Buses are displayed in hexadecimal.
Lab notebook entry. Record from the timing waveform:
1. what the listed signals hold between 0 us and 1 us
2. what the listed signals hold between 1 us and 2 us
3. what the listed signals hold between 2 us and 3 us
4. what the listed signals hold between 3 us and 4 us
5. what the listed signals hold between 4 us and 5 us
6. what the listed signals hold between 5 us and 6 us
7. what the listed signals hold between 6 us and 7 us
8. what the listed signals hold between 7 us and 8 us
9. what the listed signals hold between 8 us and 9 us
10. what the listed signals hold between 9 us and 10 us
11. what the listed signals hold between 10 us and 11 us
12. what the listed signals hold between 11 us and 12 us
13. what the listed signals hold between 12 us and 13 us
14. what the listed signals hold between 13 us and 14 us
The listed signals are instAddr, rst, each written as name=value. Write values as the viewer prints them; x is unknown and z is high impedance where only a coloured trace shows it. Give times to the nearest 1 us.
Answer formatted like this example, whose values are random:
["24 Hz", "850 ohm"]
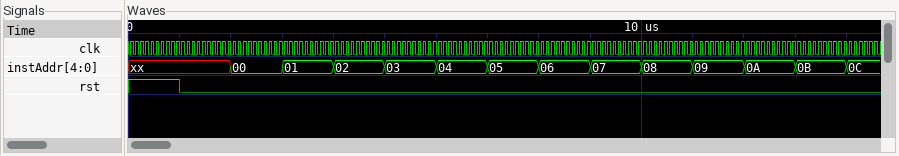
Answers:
["instAddr=xx, rst=1", "instAddr=xx, rst=0", "instAddr=00, rst=0", "instAddr=01, rst=0", "instAddr=02, rst=0", "instAddr=03, rst=0", "instAddr=04, rst=0", "instAddr=05, rst=0", "instAddr=06, rst=0", "instAddr=07, rst=0", "instAddr=08, rst=0", "instAddr=09, rst=0", "instAddr=0A, rst=0", "instAddr=0B, rst=0"]
